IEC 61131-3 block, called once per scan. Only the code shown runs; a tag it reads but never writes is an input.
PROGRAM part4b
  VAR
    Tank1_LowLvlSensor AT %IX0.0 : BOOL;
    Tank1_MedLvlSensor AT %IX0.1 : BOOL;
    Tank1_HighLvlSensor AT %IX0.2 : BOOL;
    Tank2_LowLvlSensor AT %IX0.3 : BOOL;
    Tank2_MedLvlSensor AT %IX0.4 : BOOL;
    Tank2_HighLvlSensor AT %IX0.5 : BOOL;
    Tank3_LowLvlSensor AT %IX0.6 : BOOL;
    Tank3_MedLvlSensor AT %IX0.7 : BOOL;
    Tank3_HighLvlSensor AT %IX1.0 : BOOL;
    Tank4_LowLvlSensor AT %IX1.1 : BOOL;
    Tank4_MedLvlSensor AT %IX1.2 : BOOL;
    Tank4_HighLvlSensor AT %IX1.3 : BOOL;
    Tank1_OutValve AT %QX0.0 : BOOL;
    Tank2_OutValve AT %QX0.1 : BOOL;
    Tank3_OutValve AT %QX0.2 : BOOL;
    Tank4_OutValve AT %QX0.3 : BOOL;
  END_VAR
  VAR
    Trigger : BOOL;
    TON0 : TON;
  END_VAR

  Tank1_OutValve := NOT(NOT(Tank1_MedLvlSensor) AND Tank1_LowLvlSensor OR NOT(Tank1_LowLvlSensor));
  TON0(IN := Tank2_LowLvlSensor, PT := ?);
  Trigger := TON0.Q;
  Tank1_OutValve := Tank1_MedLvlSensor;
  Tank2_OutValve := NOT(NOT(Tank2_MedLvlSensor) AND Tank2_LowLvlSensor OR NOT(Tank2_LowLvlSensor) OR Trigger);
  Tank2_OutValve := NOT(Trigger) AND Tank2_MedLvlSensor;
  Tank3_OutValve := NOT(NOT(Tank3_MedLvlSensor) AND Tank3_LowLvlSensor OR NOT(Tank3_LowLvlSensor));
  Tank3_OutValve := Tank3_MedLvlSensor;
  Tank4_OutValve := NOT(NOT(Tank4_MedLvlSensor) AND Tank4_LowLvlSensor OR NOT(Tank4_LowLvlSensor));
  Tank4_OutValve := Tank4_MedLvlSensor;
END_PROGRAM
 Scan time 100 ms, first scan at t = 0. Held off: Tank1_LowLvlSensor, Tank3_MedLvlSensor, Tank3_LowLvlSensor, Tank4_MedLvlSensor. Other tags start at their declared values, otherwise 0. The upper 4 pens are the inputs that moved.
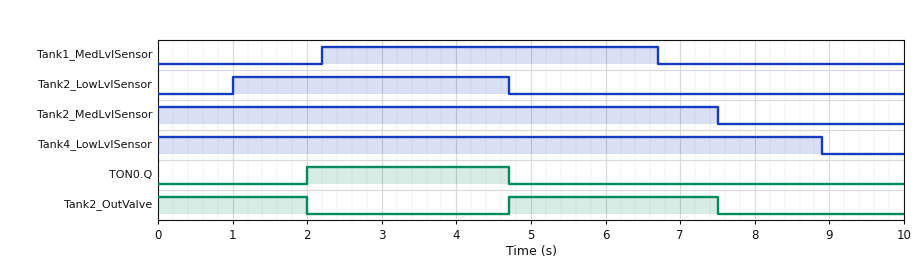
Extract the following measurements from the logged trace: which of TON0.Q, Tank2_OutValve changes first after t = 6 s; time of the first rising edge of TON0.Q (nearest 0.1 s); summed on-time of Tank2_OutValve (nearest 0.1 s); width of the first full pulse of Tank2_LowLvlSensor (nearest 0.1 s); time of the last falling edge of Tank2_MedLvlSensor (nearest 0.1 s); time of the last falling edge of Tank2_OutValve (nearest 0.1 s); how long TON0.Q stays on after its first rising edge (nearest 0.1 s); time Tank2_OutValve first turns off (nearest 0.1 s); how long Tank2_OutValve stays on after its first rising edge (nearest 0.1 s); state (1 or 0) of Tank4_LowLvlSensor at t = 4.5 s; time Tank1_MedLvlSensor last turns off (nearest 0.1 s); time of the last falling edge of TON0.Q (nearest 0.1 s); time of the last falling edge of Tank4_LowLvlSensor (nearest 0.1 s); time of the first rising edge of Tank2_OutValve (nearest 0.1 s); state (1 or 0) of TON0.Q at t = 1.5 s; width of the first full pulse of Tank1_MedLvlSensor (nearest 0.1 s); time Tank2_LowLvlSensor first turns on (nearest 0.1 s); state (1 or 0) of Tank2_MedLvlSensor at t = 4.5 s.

Tank2_OutValve
2.0 s
4.8 s
3.7 s
7.5 s
7.5 s
2.7 s
2.0 s
2.8 s
1
6.7 s
4.7 s
8.9 s
4.7 s
0
4.5 s
1.0 s
1
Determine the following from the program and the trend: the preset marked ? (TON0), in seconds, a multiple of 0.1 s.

1.0 s
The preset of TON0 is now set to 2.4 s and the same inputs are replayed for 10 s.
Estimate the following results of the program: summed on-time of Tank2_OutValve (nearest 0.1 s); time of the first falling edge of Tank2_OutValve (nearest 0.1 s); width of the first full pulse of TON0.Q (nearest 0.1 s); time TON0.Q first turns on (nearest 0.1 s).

6.2 s
3.4 s
1.3 s
3.4 s
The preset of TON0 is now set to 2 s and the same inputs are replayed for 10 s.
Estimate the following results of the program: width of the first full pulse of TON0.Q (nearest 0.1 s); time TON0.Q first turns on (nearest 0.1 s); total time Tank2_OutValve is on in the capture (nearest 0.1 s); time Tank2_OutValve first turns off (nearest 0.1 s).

1.7 s
3.0 s
5.8 s
3.0 s
